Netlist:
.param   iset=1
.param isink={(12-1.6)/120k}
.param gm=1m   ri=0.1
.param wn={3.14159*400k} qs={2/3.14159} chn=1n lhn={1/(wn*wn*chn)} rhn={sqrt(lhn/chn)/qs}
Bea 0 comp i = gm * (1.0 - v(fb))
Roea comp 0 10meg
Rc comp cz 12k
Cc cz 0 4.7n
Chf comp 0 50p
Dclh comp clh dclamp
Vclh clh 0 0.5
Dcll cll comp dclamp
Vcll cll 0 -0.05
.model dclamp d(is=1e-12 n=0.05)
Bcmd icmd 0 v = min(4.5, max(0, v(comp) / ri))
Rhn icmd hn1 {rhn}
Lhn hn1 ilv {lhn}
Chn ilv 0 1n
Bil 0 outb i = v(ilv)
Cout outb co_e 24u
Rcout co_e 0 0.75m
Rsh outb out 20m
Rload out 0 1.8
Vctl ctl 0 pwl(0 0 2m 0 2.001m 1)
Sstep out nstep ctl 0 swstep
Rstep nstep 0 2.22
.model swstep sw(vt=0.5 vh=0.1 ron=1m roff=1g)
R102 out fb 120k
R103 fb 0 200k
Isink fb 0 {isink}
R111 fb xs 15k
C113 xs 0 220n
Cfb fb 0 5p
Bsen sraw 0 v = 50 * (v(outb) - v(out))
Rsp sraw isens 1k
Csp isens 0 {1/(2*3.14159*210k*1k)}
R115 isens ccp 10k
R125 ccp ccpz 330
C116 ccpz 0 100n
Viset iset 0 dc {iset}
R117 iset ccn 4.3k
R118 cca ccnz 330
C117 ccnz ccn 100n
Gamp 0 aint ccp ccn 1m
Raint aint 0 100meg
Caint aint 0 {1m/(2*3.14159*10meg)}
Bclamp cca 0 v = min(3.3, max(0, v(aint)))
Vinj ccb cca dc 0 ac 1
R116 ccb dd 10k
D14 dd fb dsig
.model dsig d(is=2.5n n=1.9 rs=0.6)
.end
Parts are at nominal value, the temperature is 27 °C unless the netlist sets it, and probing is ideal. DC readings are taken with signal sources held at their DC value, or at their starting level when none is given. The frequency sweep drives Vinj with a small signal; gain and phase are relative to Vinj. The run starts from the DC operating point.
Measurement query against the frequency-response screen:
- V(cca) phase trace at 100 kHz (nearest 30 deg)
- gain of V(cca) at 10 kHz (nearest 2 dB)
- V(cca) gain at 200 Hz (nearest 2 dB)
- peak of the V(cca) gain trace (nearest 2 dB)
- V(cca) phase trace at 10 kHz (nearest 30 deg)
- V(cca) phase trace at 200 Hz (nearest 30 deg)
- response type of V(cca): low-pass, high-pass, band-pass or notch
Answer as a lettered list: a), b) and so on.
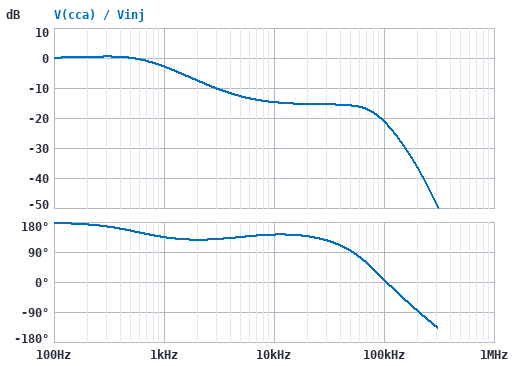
a) 0 deg
b) -14 dB
c) 0 dB
d) 0 dB
e) 150 deg
f) 180 deg
g) low-pass
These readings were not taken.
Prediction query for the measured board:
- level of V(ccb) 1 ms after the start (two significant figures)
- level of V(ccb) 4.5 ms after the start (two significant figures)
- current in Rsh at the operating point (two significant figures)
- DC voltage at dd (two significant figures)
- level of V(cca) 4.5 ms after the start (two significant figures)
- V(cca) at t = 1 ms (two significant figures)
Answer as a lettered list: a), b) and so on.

a) 2.4 V
b) 2.4 V
c) 1.0 A
d) 1.5 V
e) 2.4 V
f) 2.4 V
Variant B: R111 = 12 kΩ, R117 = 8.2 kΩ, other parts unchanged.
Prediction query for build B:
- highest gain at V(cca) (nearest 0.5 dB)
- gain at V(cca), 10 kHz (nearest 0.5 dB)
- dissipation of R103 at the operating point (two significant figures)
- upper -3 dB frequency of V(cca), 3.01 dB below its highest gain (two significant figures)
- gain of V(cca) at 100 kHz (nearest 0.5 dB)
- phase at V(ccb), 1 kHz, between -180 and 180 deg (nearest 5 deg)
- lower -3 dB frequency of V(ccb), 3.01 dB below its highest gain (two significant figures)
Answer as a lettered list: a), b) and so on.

a) 0 dB
b) -15.0 dB
c) 5.0 µW
d) 850 Hz
e) -22.5 dB
f) 40 deg
g) 1.5 kHz
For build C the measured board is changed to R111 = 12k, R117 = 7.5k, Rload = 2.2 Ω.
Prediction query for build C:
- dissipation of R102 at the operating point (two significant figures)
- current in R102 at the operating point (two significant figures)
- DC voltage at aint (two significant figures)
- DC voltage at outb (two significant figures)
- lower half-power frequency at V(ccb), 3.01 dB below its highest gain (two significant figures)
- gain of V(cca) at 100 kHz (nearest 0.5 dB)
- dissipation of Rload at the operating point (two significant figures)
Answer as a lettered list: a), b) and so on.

a) 12 µW
b) 10 µA
c) 2.3 V
d) 2.2 V
e) 1.0 kHz
f) -24.5 dB
g) 2.2 W
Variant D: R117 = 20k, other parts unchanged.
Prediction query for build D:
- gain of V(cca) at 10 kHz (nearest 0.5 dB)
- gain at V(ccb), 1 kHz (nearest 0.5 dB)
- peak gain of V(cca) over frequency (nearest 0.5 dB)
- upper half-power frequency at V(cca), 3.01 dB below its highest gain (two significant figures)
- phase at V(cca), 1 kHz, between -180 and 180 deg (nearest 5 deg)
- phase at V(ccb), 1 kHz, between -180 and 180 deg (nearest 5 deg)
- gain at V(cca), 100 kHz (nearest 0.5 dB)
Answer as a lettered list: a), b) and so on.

a) -15.0 dB
b) -3.5 dB
c) 0 dB
d) 730 Hz
e) 140 deg
f) 35 deg
g) -21.5 dB
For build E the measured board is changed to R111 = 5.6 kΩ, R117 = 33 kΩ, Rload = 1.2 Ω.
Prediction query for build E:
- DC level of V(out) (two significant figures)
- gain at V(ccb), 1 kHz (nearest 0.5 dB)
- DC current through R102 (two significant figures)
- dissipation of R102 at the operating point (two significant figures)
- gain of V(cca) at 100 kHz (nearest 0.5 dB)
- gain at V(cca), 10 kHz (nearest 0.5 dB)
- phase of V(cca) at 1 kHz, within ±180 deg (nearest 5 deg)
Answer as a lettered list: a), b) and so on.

a) 1.2 V
b) -5.5 dB
c) 1.7 µA
d) 330 nW
e) -24.0 dB
f) -13.0 dB
g) 150 deg
